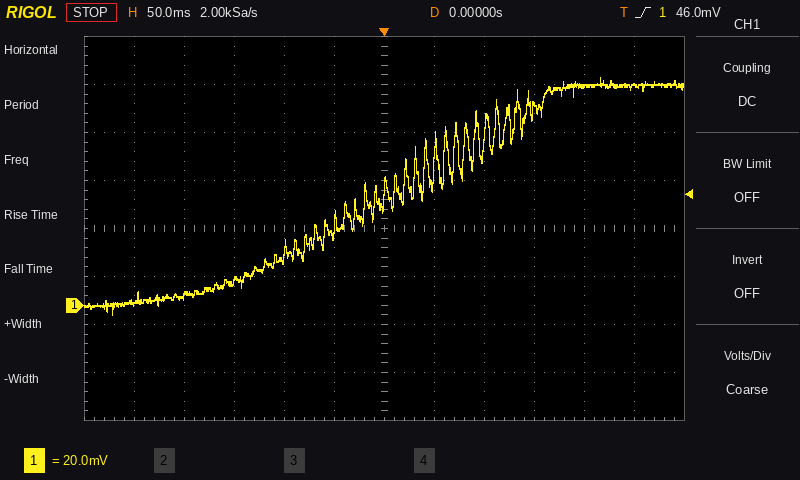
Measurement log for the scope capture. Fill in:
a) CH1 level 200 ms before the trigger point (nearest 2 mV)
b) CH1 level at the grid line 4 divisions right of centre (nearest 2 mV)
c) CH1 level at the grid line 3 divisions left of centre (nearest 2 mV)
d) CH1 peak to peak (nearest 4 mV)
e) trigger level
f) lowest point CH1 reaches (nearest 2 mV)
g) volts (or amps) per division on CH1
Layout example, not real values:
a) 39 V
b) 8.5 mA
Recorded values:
a) 4 mV
b) 92 mV
c) 10 mV
d) 100 mV
e) 46.0 mV
f) -4 mV
g) 20 mV
